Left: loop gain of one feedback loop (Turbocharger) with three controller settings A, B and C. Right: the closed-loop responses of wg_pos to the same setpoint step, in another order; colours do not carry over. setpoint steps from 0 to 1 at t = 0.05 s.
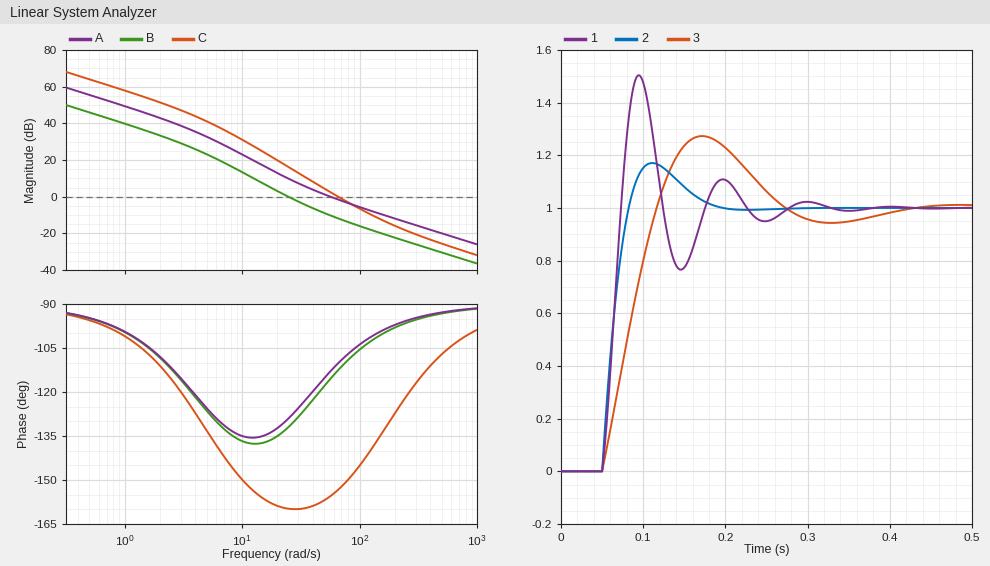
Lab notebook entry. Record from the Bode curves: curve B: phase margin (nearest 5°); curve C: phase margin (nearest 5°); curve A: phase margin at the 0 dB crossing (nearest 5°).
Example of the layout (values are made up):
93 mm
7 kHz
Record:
50°
25°
65°
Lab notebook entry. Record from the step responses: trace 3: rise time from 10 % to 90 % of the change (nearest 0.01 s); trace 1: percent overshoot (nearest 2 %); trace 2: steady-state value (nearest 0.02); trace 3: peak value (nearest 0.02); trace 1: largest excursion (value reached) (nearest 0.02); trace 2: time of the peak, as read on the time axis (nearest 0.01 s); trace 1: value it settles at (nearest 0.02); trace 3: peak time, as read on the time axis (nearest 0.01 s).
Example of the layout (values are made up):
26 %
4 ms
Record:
0.05 s
50 %
1.00
1.28
1.50
0.11 s
1.00
0.17 s
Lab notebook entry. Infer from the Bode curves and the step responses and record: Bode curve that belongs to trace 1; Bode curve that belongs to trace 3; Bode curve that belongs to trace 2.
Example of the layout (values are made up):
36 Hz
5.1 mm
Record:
C
B
A
